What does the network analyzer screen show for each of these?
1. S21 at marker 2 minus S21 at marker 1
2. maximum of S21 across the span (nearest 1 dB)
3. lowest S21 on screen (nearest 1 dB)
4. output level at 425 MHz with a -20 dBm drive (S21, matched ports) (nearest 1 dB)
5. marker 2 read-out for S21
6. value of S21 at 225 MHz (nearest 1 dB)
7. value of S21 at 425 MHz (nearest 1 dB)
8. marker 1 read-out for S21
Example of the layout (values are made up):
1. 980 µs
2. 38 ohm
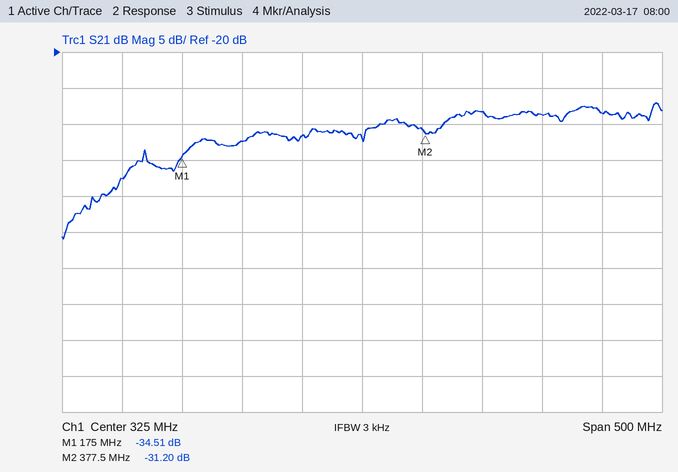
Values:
1. 3.31 dB
2. -27 dB
3. -46 dB
4. -48 dBm
5. -31.20 dB
6. -32 dB
7. -28 dB
8. -34.51 dB
